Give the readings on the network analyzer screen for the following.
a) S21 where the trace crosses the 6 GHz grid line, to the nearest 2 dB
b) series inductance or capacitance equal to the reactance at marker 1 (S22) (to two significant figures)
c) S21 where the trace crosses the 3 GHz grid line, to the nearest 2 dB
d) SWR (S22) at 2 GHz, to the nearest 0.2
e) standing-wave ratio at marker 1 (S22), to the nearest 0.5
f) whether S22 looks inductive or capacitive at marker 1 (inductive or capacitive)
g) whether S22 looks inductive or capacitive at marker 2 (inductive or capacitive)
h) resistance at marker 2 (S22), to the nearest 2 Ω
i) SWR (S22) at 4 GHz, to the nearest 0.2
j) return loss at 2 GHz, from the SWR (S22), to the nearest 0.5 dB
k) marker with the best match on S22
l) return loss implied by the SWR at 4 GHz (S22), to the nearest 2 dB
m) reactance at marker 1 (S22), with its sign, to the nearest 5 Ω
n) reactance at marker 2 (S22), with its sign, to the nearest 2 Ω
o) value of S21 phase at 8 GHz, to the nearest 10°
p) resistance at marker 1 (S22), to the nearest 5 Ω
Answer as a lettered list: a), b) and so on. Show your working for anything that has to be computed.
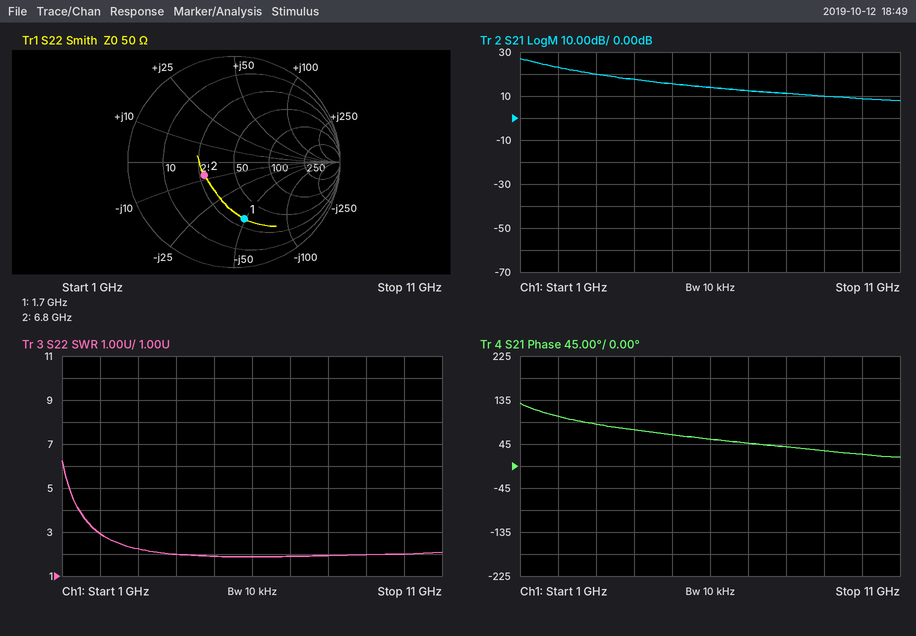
a) 14 dB
b) C = 1/(2π × 1.7 GHz × 50 Ω) ≈ 1.9 pF
c) 20 dB
d) 3.0
e) 3.5
f) capacitive
g) capacitive
h) 28 Ω
i) 2.0
j) −20 log10((3 − 1)/(3 + 1)) ≈ 6.0 dB
k) marker 2
l) −20 log10((2 − 1)/(2 + 1)) ≈ 10 dB
m) -50 Ω
n) -8 Ω
o) 40°
p) 30 Ω
